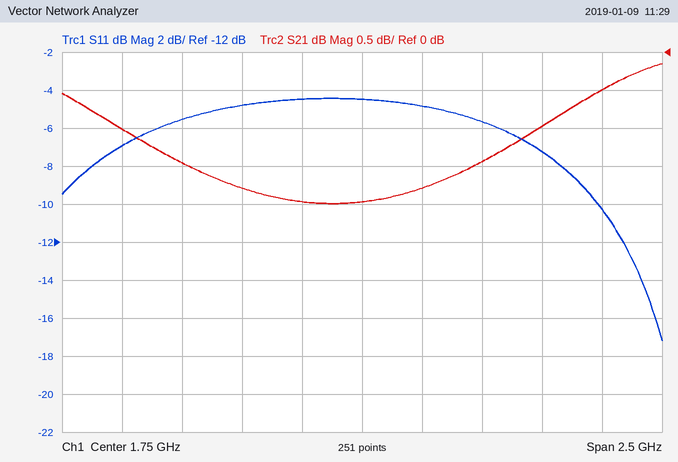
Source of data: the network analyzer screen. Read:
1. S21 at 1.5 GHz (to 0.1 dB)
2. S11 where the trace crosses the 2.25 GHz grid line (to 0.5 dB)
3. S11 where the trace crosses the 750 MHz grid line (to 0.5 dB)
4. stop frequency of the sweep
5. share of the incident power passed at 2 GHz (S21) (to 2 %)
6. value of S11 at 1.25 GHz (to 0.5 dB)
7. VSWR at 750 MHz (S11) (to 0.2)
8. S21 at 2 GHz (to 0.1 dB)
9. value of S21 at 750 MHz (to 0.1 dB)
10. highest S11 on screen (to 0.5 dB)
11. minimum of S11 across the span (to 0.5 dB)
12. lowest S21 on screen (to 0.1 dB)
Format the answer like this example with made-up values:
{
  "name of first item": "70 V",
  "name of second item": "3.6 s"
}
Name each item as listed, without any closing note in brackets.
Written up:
{
  "S21 at 1.5 GHz": "-2.0 dB",
  "S11 where the trace crosses the 2.25 GHz grid line": "-5.5 dB",
  "S11 where the trace crosses the 750 MHz grid line": "-7.0 dB",
  "stop frequency of the sweep": "3 GHz",
  "share of the incident power passed at 2 GHz (S21)": "66 %",
  "value of S11 at 1.25 GHz": "-5.0 dB",
  "VSWR at 750 MHz (S11)": "2.6",
  "S21 at 2 GHz": "-1.8 dB",
  "value of S21 at 750 MHz": "-1.0 dB",
  "highest S11 on screen": "-4.5 dB",
  "minimum of S11 across the span": "-17.0 dB",
  "lowest S21 on screen": "-2.0 dB"
}
